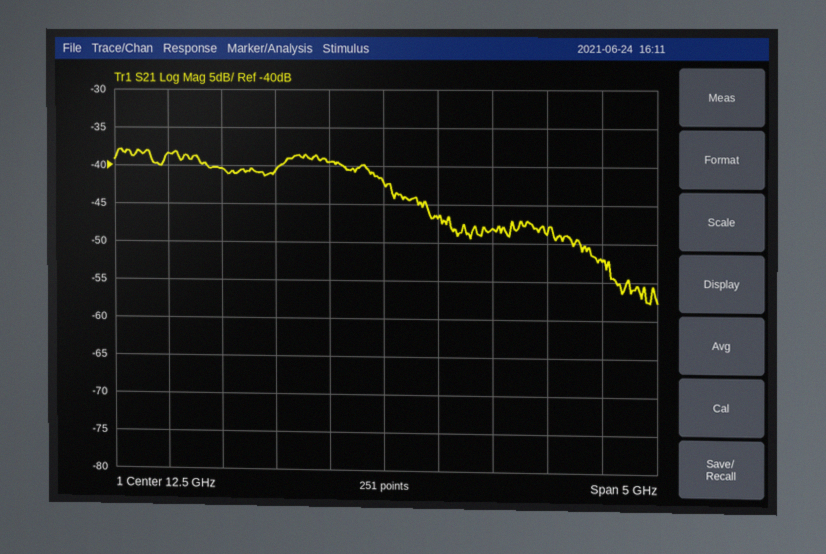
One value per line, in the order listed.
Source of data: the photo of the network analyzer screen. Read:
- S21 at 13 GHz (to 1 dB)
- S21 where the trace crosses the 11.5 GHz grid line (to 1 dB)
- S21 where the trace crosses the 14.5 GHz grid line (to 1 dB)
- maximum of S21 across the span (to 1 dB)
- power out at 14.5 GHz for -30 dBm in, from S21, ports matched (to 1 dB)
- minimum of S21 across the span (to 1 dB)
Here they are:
-47 dB
-41 dB
-52 dB
-38 dB
-82 dBm
-58 dB
